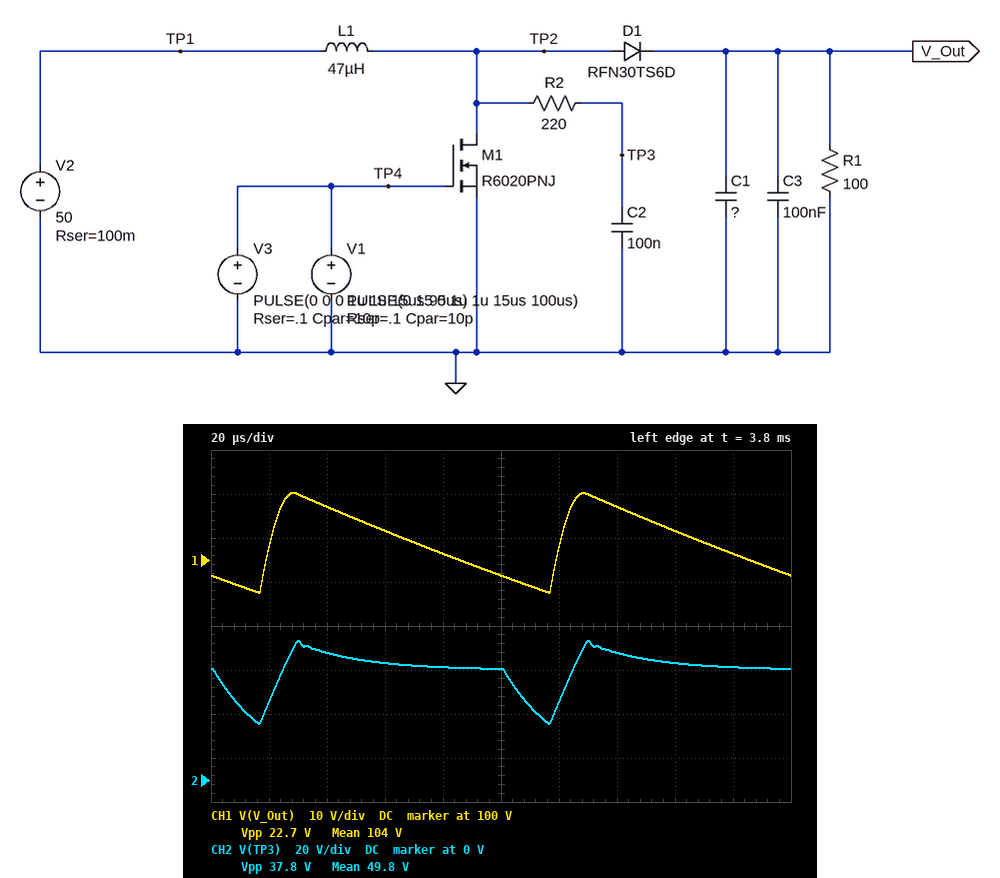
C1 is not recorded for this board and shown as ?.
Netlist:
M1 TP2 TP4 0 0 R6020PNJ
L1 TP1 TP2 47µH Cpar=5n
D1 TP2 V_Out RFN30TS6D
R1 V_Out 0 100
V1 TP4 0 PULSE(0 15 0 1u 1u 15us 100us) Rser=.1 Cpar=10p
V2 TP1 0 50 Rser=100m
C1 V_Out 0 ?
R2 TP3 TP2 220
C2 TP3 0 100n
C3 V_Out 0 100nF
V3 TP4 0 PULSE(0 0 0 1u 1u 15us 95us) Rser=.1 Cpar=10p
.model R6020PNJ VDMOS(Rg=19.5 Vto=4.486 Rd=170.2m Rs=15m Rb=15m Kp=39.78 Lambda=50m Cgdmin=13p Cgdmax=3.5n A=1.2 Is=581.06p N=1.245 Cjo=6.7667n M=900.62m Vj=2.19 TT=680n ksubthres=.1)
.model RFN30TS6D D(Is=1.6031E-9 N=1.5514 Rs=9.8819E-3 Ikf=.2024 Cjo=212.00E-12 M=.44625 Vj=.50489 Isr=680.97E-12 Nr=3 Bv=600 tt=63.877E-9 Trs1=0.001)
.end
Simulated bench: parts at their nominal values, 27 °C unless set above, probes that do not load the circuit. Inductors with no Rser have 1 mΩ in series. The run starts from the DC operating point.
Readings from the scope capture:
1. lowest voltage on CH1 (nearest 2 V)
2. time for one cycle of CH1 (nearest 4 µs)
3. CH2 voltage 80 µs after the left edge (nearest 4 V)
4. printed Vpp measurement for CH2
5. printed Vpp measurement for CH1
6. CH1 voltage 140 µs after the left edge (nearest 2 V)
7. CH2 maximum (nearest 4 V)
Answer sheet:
92 V
100 µs
52 V
37.8 V
22.7 V
112 V
64 V
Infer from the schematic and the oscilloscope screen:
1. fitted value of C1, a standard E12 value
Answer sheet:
3.9 µF
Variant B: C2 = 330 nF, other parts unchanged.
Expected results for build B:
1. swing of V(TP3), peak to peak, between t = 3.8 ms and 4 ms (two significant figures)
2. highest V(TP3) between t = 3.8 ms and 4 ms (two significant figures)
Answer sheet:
11 V
52 V
